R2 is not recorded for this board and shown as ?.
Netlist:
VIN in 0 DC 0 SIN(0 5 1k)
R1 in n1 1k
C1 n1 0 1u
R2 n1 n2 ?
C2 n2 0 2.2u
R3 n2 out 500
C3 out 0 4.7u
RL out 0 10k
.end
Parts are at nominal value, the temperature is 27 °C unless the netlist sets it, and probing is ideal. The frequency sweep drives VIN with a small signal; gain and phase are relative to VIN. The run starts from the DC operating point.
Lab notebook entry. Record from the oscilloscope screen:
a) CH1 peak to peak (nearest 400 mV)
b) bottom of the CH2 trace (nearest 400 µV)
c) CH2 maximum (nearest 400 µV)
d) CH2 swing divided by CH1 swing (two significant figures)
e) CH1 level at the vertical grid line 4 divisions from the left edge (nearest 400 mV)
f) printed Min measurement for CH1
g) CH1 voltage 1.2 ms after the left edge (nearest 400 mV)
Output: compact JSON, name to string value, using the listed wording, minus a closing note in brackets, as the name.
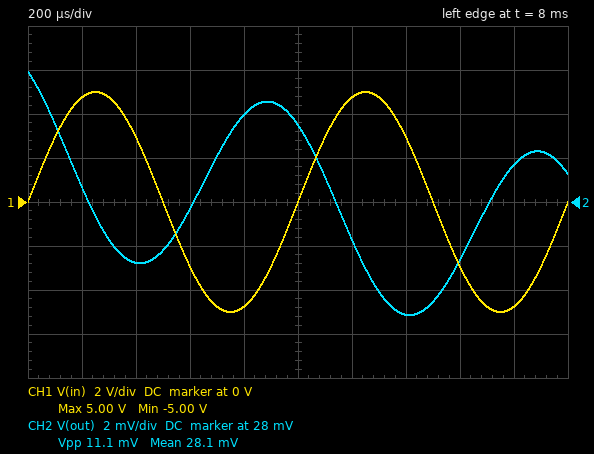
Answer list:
{"CH1 peak to peak": "10.0 V", "bottom of the CH2 trace": "22.8 mV", "CH2 maximum": "34.0 mV", "CH2 swing divided by CH1 swing": "0.0011", "CH1 level at the vertical grid line 4 divisions from the left edge": "-4.8 V", "printed Min measurement for CH1": "-5.00 V", "CH1 voltage 1.2 ms after the left edge": "4.8 V"}
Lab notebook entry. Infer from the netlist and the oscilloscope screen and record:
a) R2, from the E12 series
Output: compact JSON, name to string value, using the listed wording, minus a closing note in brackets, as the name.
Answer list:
{"R2, from the E12 series": "820 Ω"}
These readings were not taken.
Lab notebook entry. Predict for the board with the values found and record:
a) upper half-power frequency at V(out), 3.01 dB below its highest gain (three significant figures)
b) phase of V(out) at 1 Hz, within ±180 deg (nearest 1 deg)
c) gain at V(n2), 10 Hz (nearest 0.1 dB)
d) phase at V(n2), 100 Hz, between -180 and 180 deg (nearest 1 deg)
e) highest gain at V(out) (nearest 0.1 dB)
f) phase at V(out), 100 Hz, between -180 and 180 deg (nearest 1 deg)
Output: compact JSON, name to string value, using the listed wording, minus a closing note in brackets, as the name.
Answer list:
{"upper half-power frequency at V(out), 3.01 dB below its highest gain": "13.2 Hz", "phase of V(out) at 1 Hz, within ±180 deg": "-5 deg", "gain at V(n2), 10 Hz": "-3.3 dB", "phase at V(n2), 100 Hz, between -180 and 180 deg": "-67 deg", "highest gain at V(out)": "-1.8 dB", "phase at V(out), 100 Hz, between -180 and 180 deg": "-122 deg"}
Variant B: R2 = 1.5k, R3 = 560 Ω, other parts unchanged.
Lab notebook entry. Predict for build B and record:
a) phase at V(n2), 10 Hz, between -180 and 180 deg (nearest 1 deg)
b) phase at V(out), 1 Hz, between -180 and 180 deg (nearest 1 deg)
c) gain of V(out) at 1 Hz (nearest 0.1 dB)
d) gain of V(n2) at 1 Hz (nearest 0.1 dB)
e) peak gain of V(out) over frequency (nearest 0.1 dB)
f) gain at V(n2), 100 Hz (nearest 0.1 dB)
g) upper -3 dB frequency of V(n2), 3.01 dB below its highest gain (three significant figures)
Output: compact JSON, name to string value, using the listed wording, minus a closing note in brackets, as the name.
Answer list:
{"phase at V(n2), 10 Hz, between -180 and 180 deg": "-39 deg", "phase at V(out), 1 Hz, between -180 and 180 deg": "-6 deg", "gain of V(out) at 1 Hz": "-2.4 dB", "gain of V(n2) at 1 Hz": "-1.9 dB", "peak gain of V(out) over frequency": "-2.3 dB", "gain at V(n2), 100 Hz": "-17.6 dB", "upper -3 dB frequency of V(n2), 3.01 dB below its highest gain": "10.9 Hz"}
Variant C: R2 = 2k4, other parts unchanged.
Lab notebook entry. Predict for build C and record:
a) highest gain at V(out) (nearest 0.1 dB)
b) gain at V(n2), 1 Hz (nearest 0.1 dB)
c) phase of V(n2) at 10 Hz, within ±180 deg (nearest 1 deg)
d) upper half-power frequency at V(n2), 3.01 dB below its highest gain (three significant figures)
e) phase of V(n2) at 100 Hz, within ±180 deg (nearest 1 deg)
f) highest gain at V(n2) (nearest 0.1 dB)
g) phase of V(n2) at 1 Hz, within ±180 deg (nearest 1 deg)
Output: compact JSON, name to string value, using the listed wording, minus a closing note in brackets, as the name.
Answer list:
{"highest gain at V(out)": "-2.9 dB", "gain at V(n2), 1 Hz": "-2.5 dB", "phase of V(n2) at 10 Hz, within ±180 deg": "-46 deg", "upper half-power frequency at V(n2), 3.01 dB below its highest gain": "8.78 Hz", "phase of V(n2) at 100 Hz, within ±180 deg": "-78 deg", "highest gain at V(n2)": "-2.4 dB", "phase of V(n2) at 1 Hz, within ±180 deg": "-6 deg"}
